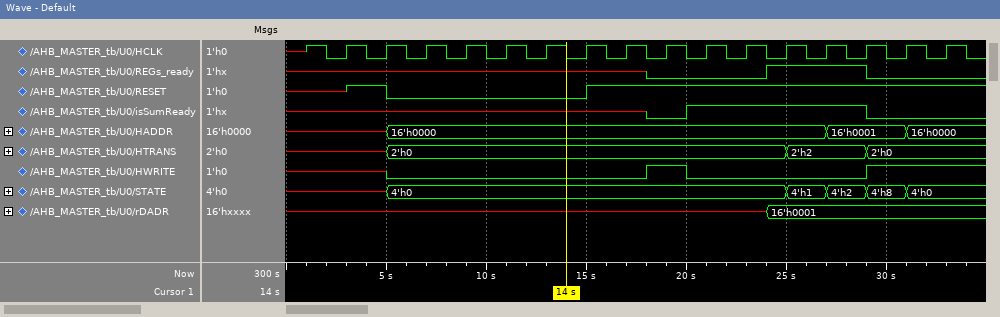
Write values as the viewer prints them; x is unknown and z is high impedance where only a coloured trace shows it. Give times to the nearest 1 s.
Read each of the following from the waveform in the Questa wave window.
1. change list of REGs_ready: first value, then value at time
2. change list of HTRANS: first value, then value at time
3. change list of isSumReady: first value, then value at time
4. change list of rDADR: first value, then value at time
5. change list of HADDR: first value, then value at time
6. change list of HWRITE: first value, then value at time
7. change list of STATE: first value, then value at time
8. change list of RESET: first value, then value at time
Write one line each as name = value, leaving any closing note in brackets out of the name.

change list of REGs_ready: first value, then value at time = x, 0 at 18 s, 1 at 24 s, 0 at 29 s
change list of HTRANS: first value, then value at time = x, 2'h0 at 5 s, 2'h2 at 25 s, 2'h0 at 29 s
change list of isSumReady: first value, then value at time = x, 0 at 18 s, 1 at 20 s, 0 at 29 s
change list of rDADR: first value, then value at time = x, 16'h0001 at 24 s
change list of HADDR: first value, then value at time = x, 16'h0000 at 5 s, 16'h0001 at 27 s, 16'h0000 at 31 s
change list of HWRITE: first value, then value at time = x, 0 at 5 s, 1 at 18 s, 0 at 20 s, 1 at 29 s
change list of STATE: first value, then value at time = x, 4'h0 at 5 s, 4'h1 at 25 s, 4'h2 at 27 s, 4'h8 at 29 s, 4'h0 at 31 s
change list of RESET: first value, then value at time = x, 1 at 3 s, 0 at 5 s, 1 at 15 s
